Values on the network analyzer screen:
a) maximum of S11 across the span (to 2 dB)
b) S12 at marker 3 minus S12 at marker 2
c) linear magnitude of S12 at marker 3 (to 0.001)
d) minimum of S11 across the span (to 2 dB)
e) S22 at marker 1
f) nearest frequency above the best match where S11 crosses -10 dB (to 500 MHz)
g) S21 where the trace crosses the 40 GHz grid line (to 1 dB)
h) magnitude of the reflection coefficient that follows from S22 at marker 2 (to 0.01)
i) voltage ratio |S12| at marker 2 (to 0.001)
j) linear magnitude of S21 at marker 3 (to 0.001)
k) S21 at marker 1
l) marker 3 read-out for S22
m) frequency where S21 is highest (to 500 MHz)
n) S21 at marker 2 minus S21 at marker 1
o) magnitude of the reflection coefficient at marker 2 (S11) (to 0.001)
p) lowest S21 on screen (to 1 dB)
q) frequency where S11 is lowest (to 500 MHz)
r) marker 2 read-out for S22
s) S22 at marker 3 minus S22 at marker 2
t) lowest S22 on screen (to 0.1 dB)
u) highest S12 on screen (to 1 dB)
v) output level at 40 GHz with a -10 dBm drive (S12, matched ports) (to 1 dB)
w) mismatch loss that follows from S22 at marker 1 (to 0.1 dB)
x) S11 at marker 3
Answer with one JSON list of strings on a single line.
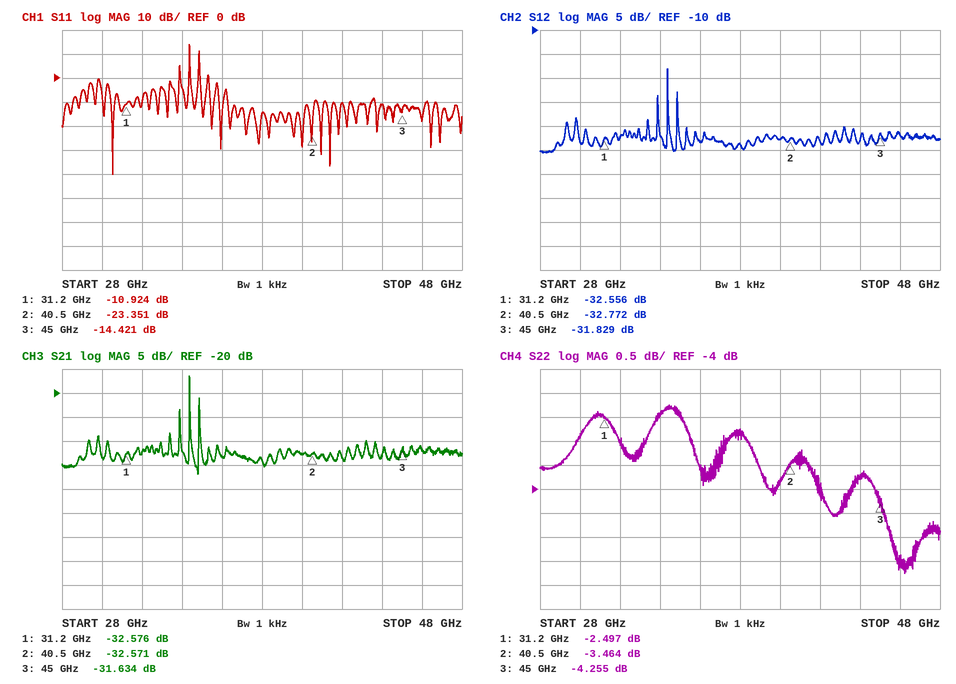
["14 dB", "0.943 dB", "0.026", "-40 dB", "-2.497 dB", "30.5 GHz", "-33 dB", "0.67", "0.023", "0.026", "-32.576 dB", "-4.255 dB", "34.5 GHz", "0.005 dB", "0.068", "-37 dB", "30.5 GHz", "-3.464 dB", "-0.791 dB", "-5.8 dB", "-18 dB", "-43 dBm", "3.6 dB", "-14.421 dB"]
